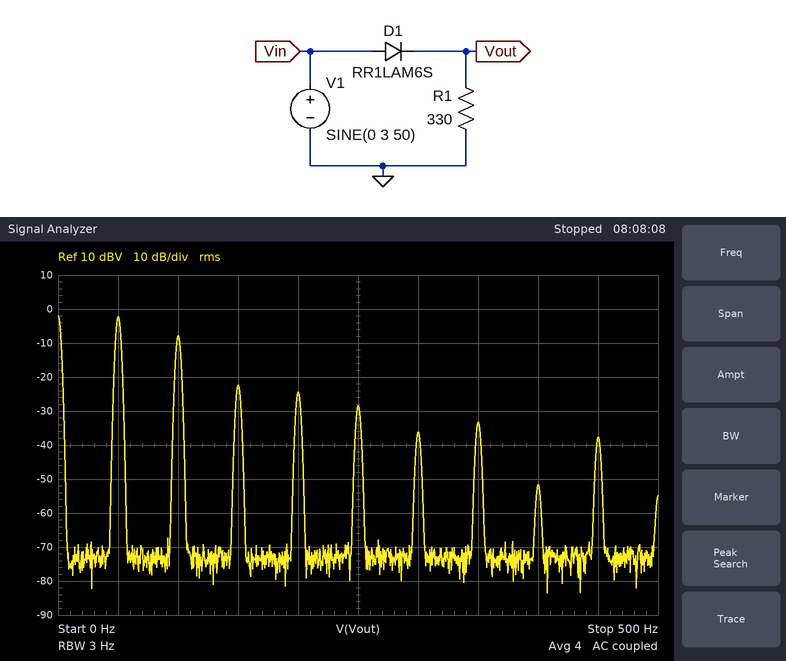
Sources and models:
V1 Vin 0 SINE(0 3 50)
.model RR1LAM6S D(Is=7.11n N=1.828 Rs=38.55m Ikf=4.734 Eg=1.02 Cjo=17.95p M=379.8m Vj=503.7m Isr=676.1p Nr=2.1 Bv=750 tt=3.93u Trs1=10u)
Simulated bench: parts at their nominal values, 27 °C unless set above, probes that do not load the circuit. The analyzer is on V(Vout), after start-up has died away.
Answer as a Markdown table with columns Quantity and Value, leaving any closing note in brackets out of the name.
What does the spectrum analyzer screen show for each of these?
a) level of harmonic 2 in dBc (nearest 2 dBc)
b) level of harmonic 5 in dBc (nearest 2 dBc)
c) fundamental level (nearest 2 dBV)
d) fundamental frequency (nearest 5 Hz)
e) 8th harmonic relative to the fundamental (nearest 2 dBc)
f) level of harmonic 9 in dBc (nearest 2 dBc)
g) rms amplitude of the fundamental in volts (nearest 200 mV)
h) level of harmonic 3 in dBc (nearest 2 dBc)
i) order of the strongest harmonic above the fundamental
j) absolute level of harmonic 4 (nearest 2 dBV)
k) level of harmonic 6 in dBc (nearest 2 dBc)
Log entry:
| Quantity | Value |
|---|---|
| level of harmonic 2 in dBc | -6 dBc |
| level of harmonic 5 in dBc | -26 dBc |
| fundamental level | -2 dBV |
| fundamental frequency | 50 Hz |
| 8th harmonic relative to the fundamental | -50 dBc |
| level of harmonic 9 in dBc | -36 dBc |
| rms amplitude of the fundamental in volts | 800 mV |
| level of harmonic 3 in dBc | -20 dBc |
| order of the strongest harmonic above the fundamental | 2 |
| absolute level of harmonic 4 | -24 dBV |
| level of harmonic 6 in dBc | -34 dBc |
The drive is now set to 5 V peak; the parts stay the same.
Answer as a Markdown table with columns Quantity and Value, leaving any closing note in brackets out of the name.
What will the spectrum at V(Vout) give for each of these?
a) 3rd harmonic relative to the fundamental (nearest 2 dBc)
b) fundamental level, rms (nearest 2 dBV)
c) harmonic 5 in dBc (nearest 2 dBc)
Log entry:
| Quantity | Value |
|---|---|
| 3rd harmonic relative to the fundamental | -24 dBc |
| fundamental level, rms | 4 dBV |
| harmonic 5 in dBc | -30 dBc |
